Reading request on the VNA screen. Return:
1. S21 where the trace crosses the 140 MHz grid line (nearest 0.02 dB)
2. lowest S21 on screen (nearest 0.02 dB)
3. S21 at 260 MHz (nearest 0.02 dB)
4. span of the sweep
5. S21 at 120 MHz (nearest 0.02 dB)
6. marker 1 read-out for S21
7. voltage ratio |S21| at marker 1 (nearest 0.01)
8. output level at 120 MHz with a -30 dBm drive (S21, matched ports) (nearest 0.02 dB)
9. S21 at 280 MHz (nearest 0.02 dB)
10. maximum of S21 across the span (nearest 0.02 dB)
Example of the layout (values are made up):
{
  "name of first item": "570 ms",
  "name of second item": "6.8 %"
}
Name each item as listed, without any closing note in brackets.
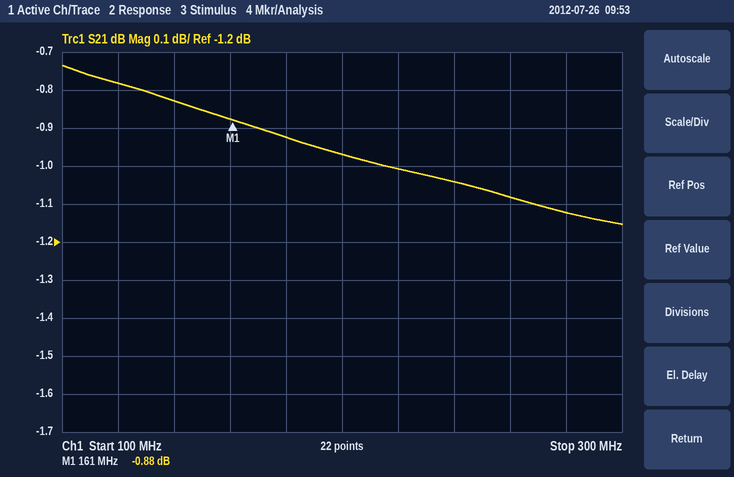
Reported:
{
  "S21 where the trace crosses the 140 MHz grid line": "-0.82 dB",
  "lowest S21 on screen": "-1.16 dB",
  "S21 at 260 MHz": "-1.08 dB",
  "span of the sweep": "200 MHz",
  "S21 at 120 MHz": "-0.78 dB",
  "marker 1 read-out for S21": "-0.88 dB",
  "voltage ratio |S21| at marker 1": "0.90",
  "output level at 120 MHz with a -30 dBm drive (S21, matched ports)": "-30.78 dBm",
  "S21 at 280 MHz": "-1.12 dB",
  "maximum of S21 across the span": "-0.74 dB"
}
